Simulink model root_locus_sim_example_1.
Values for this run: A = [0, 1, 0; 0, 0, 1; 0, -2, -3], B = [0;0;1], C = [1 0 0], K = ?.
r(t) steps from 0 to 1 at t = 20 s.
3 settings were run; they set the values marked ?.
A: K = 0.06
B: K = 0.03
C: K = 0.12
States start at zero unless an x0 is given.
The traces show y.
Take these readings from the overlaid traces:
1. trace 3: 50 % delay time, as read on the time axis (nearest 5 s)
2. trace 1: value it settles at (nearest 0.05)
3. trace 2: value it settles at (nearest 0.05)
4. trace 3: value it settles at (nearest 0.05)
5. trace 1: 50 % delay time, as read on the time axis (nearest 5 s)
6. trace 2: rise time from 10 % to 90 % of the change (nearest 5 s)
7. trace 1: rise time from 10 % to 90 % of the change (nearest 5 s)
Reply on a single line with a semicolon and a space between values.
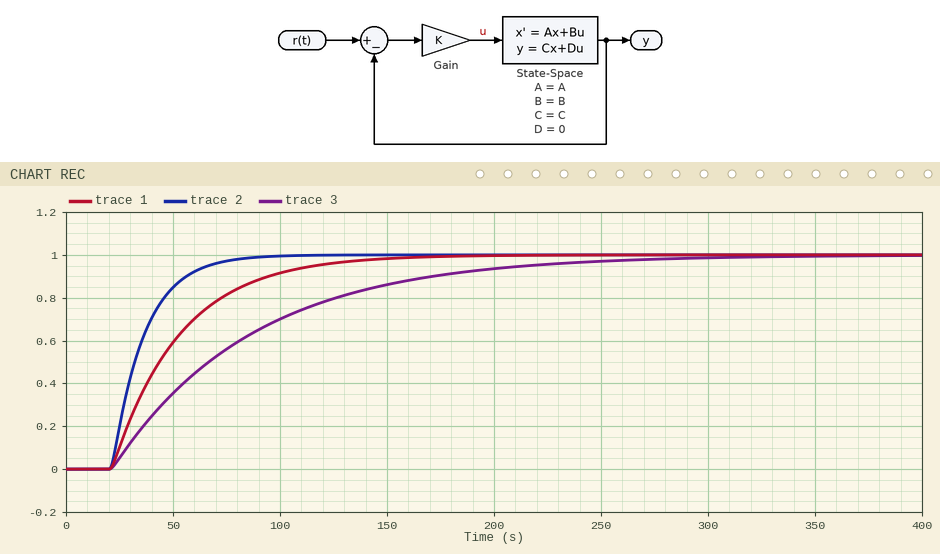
65 s; 1.00; 1.00; 1.00; 45 s; 35 s; 70 s
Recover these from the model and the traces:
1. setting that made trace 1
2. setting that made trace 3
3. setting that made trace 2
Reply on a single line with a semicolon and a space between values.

A; B; C
